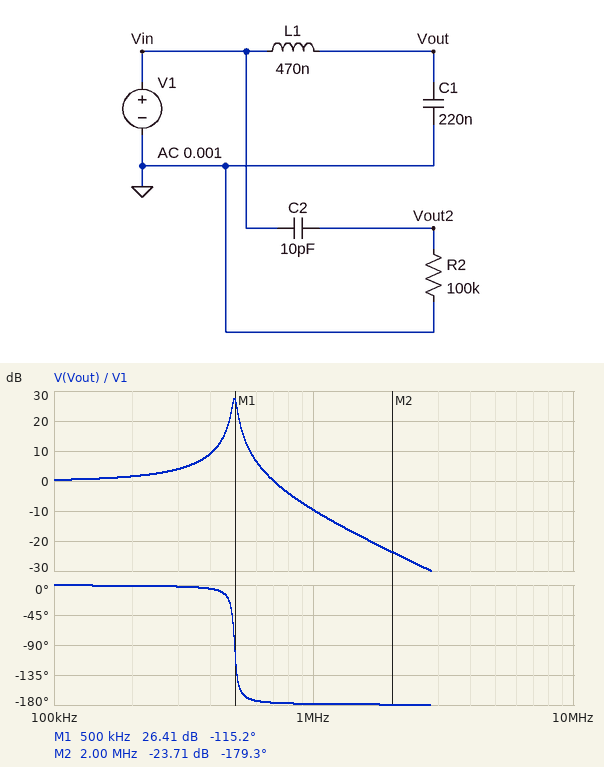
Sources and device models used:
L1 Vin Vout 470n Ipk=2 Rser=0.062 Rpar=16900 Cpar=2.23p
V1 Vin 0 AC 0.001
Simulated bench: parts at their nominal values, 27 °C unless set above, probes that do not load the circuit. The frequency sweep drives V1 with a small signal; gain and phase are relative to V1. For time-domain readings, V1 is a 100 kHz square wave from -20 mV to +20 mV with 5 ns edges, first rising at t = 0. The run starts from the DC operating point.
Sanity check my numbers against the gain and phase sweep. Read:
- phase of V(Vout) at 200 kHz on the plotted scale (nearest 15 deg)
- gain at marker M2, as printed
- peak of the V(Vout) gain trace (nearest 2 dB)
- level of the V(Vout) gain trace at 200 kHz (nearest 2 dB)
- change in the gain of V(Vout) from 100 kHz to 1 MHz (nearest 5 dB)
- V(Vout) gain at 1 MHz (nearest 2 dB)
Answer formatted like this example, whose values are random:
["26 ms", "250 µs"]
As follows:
["0 deg", "-23.71 dB", "28 dB", "2 dB", "-10 dB", "-10 dB"]
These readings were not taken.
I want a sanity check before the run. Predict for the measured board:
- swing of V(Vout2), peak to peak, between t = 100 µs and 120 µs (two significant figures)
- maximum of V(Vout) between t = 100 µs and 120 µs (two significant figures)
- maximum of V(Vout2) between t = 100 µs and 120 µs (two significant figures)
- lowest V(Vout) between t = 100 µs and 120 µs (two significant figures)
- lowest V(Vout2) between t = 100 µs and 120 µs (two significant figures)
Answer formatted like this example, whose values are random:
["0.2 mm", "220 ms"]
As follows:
["79 mV", "140 mV", "40 mV", "-140 mV", "-40 mV"]
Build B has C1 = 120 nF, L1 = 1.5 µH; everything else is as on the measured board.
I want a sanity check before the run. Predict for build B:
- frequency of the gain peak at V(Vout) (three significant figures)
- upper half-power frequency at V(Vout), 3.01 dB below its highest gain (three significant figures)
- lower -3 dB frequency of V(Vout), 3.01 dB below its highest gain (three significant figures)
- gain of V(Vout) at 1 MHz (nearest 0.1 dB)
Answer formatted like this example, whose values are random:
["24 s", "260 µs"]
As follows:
["375 kHz", "378 kHz", "372 kHz", "-15.7 dB"]
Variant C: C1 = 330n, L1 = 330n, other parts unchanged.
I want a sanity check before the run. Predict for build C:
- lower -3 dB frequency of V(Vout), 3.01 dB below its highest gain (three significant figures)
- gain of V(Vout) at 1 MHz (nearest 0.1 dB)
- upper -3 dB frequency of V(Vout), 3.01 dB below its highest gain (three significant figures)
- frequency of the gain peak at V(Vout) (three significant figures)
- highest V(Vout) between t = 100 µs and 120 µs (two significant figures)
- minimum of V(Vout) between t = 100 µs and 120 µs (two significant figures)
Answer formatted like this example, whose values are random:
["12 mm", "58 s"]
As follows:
["467 kHz", "-10.4 dB", "497 kHz", "482 kHz", "81 mV", "-81 mV"]
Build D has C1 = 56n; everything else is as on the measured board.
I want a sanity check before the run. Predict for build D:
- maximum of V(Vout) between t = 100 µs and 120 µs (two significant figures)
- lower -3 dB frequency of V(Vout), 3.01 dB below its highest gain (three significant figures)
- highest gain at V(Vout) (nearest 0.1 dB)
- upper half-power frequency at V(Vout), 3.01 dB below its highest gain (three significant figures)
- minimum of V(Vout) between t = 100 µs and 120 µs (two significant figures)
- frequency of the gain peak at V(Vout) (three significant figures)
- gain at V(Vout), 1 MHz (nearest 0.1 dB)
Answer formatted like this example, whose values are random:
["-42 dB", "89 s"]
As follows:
["44 mV", "970 kHz", "33.3 dB", "991 kHz", "-44 mV", "981 kHz", "27.0 dB"]
